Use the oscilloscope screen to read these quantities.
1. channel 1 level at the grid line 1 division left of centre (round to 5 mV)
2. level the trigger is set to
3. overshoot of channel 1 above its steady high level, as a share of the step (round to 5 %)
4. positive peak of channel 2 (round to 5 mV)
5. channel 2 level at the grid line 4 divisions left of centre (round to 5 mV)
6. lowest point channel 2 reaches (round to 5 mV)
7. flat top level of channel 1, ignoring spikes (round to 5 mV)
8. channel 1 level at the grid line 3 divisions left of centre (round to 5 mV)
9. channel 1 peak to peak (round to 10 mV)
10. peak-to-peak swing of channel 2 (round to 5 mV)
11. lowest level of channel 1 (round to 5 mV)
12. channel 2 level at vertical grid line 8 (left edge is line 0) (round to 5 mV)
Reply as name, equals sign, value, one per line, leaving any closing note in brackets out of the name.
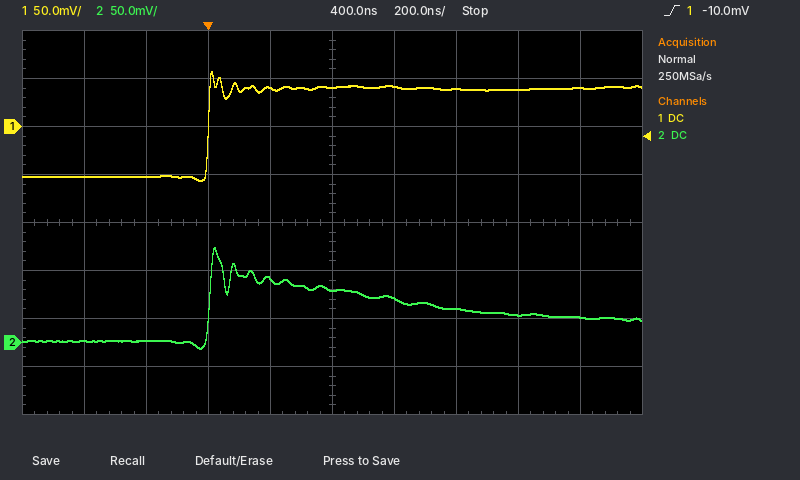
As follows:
channel 1 level at the grid line 1 division left of centre = 40 mV
level the trigger is set to = -10.0 mV
overshoot of channel 1 above its steady high level, as a share of the step = 20 %
positive peak of channel 2 = 100 mV
channel 2 level at the grid line 4 divisions left of centre = 0 mV
lowest point channel 2 reaches = -5 mV
flat top level of channel 1, ignoring spikes = 40 mV
channel 1 level at the grid line 3 divisions left of centre = -50 mV
channel 1 peak to peak = 110 mV
peak-to-peak swing of channel 2 = 105 mV
lowest level of channel 1 = -55 mV
channel 2 level at vertical grid line 8 (left edge is line 0) = 30 mV
